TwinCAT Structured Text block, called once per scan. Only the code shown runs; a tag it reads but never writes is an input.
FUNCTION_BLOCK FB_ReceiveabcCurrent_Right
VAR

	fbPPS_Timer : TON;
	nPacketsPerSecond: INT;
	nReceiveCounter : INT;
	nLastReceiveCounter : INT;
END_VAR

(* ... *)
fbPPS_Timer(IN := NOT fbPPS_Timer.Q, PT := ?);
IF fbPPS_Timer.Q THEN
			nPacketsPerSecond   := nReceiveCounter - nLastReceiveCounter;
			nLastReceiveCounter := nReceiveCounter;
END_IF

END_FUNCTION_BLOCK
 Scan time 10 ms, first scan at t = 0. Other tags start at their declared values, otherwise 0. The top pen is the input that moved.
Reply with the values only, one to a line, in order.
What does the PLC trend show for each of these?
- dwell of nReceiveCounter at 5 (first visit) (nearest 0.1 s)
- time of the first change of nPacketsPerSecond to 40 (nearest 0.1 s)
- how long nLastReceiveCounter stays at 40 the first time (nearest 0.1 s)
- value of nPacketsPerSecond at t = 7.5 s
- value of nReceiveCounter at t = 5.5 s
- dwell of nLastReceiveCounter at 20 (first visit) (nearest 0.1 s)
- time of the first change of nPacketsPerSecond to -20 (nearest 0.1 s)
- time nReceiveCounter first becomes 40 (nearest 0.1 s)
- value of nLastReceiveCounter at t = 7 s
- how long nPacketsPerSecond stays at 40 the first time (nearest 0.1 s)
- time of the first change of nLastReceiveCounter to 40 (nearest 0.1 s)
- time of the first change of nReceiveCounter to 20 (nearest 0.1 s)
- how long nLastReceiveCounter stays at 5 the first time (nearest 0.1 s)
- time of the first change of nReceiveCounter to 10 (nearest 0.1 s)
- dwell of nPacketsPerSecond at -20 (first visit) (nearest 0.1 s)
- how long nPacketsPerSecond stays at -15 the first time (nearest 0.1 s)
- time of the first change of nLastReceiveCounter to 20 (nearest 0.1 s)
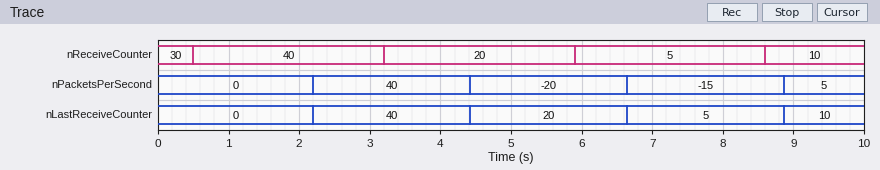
2.7 s
2.2 s
2.2 s
-15
20
2.2 s
4.4 s
0.5 s
5
2.2 s
2.2 s
3.2 s
2.2 s
8.6 s
2.2 s
2.2 s
4.4 s
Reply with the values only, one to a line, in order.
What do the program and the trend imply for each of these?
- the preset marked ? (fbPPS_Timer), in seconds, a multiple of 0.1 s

2.2 s
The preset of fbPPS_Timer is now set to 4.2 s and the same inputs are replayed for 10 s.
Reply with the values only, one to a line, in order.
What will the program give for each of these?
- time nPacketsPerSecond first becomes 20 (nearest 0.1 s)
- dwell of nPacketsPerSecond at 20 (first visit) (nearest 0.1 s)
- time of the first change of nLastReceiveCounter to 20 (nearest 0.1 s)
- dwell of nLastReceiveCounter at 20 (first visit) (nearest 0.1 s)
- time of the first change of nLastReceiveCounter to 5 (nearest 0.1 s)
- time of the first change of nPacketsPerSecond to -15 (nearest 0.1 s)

4.2 s
4.2 s
4.2 s
4.2 s
8.4 s
8.4 s
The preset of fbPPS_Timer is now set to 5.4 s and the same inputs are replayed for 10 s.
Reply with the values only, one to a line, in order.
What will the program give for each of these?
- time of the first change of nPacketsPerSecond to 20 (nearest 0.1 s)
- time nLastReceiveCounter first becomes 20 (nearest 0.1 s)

5.4 s
5.4 s
